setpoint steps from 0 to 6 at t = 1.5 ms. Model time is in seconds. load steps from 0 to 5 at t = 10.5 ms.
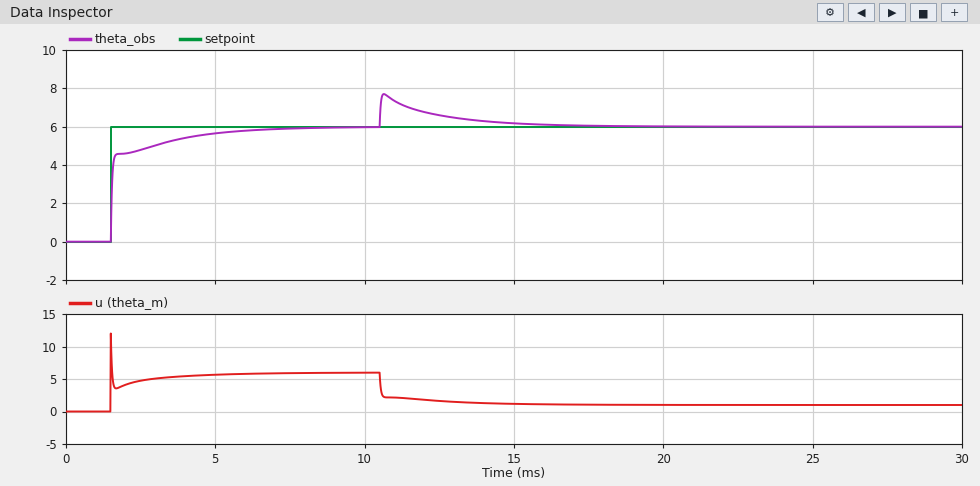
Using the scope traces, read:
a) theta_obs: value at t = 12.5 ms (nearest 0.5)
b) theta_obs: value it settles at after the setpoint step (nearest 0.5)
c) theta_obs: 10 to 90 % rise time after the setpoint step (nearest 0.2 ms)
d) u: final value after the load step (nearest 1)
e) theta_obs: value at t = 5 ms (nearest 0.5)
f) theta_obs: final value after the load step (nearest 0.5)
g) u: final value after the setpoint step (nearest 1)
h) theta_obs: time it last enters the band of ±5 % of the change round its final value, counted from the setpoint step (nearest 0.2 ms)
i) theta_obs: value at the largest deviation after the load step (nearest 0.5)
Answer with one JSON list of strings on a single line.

["6.5", "6.0", "2.4 ms", "1", "5.5", "6.0", "6", "3.8 ms", "7.5"]
